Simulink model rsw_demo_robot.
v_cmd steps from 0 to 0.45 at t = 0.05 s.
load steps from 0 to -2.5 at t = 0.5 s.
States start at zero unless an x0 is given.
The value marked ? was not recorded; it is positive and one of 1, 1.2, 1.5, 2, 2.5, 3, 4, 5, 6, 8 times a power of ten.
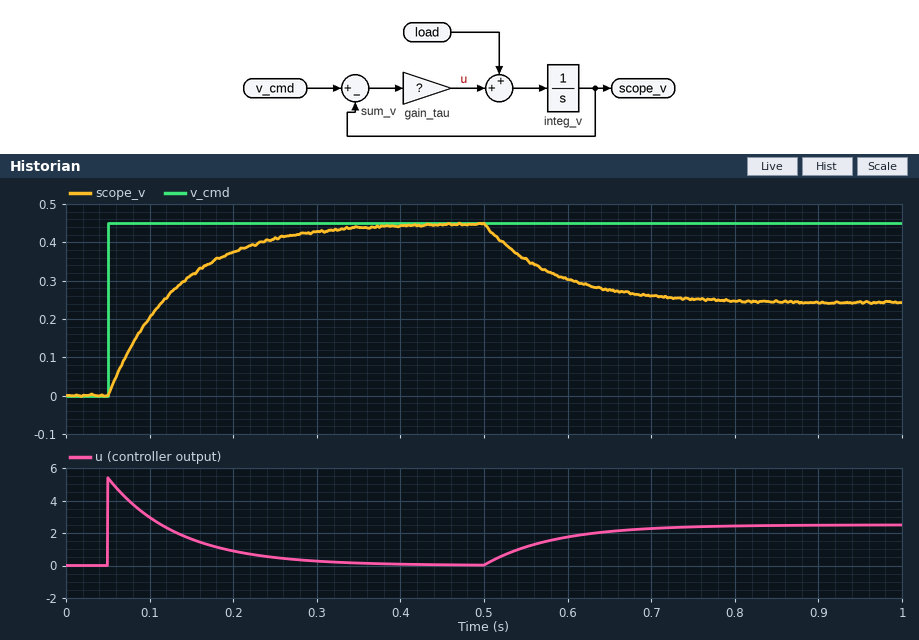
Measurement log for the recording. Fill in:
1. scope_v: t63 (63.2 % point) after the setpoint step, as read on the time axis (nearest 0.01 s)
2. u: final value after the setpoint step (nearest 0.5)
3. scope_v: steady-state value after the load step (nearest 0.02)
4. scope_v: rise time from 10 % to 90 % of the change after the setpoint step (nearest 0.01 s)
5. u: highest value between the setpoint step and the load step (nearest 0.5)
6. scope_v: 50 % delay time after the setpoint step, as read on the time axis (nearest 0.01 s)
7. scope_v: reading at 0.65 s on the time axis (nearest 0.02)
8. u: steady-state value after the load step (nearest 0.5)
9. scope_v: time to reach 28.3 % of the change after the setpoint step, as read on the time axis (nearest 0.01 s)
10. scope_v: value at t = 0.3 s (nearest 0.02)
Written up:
0.13 s
0.0
0.24
0.18 s
5.5
0.11 s
0.28
2.5
0.08 s
0.42
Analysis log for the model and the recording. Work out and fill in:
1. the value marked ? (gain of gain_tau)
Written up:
12
